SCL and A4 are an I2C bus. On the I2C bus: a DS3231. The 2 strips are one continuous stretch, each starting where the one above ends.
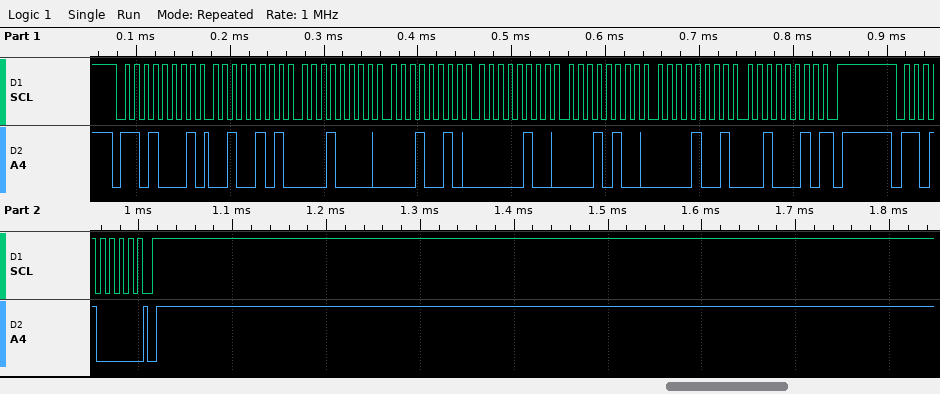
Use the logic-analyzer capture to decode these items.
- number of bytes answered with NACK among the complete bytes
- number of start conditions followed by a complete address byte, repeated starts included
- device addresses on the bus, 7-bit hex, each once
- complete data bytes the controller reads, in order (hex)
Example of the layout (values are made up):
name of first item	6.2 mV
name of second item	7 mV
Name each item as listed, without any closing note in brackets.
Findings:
number of bytes answered with NACK among the complete bytes	1
number of start conditions followed by a complete address byte, repeated starts included	2
device addresses on the bus, 7-bit hex, each once	0x68
complete data bytes the controller reads, in order	25 10 12 04 14 09 22
